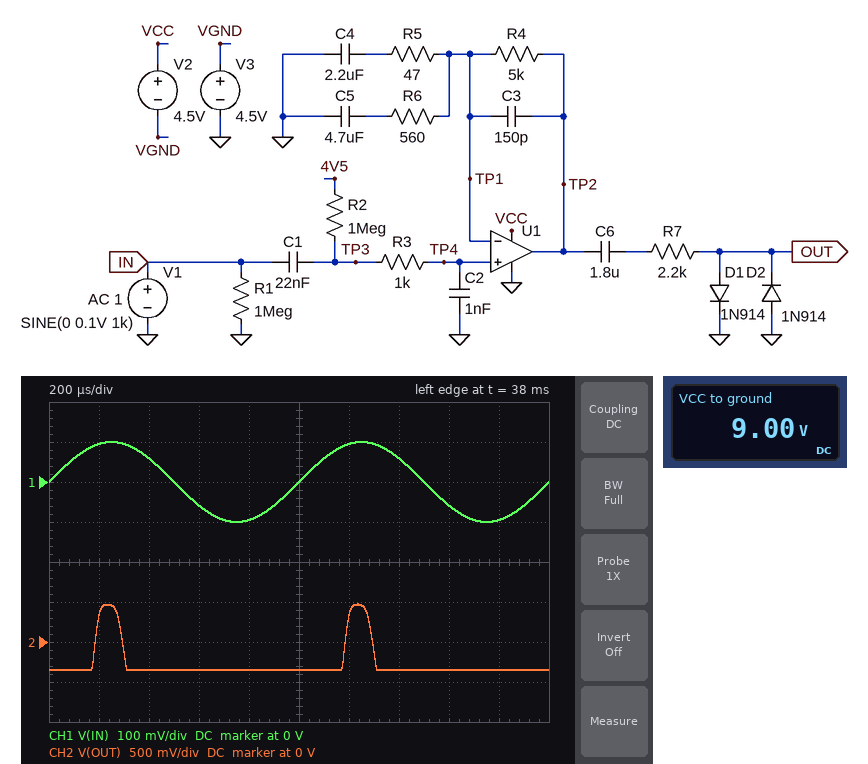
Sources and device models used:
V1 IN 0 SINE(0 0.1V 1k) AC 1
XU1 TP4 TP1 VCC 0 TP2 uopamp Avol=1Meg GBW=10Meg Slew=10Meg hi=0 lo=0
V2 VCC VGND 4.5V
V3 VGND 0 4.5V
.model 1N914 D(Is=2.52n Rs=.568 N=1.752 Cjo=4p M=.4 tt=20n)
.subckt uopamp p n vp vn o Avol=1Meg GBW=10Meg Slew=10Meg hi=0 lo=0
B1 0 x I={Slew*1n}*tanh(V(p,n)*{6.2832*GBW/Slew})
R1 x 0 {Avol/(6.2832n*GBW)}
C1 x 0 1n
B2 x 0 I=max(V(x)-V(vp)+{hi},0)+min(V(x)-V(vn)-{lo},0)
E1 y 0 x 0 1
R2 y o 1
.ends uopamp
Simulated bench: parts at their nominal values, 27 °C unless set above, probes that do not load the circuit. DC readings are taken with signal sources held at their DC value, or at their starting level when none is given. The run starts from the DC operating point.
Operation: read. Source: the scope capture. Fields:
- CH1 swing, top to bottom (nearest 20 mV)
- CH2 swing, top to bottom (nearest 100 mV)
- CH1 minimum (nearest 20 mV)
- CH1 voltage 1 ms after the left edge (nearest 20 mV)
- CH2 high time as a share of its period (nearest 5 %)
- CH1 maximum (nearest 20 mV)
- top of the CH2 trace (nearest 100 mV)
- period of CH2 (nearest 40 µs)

200 mV
800 mV
-100 mV
0 V
10 %
100 mV
500 mV
1.00 ms
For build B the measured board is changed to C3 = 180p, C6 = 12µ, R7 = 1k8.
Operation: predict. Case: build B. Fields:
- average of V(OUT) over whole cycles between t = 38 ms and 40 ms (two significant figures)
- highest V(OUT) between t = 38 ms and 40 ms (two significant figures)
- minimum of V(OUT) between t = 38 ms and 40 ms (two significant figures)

-78 mV
510 mV
-150 mV
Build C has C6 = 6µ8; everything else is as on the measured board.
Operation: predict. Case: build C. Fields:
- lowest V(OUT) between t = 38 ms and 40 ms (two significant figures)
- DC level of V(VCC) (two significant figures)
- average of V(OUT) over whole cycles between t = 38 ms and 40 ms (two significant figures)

-210 mV
9.0 V
-130 mV
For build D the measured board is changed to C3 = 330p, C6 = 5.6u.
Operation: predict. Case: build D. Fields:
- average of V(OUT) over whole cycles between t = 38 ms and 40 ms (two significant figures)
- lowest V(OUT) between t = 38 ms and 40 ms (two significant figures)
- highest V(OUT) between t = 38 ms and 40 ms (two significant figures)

-160 mV
-240 mV
490 mV
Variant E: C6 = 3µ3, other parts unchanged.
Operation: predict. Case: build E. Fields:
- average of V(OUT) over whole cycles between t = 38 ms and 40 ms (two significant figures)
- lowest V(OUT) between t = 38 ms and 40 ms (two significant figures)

-240 mV
-330 mV
